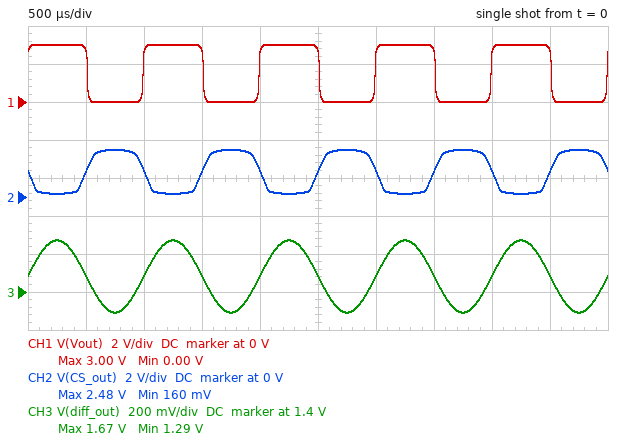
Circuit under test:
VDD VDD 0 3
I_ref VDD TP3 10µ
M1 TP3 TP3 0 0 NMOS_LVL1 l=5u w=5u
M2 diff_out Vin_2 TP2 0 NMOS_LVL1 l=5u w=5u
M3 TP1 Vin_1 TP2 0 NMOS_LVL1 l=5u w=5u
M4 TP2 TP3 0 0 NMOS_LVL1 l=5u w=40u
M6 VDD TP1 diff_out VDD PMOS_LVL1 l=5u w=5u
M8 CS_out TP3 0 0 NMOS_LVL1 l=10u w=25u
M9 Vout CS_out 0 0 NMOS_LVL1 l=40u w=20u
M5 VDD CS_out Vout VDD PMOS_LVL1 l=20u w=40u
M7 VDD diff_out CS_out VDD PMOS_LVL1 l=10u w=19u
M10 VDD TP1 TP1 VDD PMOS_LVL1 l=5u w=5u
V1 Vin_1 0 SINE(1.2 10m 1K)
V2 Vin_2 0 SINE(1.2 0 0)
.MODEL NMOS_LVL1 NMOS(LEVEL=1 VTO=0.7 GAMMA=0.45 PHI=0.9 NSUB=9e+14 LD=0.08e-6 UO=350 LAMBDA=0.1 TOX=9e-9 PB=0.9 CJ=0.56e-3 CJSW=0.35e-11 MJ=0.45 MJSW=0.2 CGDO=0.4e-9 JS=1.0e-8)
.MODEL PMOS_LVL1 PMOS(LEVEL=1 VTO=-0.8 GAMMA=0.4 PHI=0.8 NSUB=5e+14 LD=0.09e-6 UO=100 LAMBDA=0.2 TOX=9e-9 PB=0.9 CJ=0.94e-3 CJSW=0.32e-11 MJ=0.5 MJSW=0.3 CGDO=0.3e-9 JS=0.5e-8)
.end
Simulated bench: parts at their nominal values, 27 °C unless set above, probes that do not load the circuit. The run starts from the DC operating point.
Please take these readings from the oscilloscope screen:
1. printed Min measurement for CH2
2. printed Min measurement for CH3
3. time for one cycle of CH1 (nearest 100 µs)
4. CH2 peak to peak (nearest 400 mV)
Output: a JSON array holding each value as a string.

["160 mV", "1.29 V", "1.0 ms", "2.4 V"]
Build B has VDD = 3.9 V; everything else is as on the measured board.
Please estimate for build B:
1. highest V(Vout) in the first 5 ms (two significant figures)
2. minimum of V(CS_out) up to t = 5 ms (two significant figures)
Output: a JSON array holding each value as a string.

["3.9 V", "210 mV"]
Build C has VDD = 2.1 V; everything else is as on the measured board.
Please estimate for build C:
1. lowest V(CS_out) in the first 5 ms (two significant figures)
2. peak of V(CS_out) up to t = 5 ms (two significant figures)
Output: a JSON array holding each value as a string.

["140 mV", "1.6 V"]
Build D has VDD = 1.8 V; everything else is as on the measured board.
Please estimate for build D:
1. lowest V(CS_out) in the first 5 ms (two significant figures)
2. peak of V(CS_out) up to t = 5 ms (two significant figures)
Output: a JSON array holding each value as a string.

["250 mV", "290 mV"]
